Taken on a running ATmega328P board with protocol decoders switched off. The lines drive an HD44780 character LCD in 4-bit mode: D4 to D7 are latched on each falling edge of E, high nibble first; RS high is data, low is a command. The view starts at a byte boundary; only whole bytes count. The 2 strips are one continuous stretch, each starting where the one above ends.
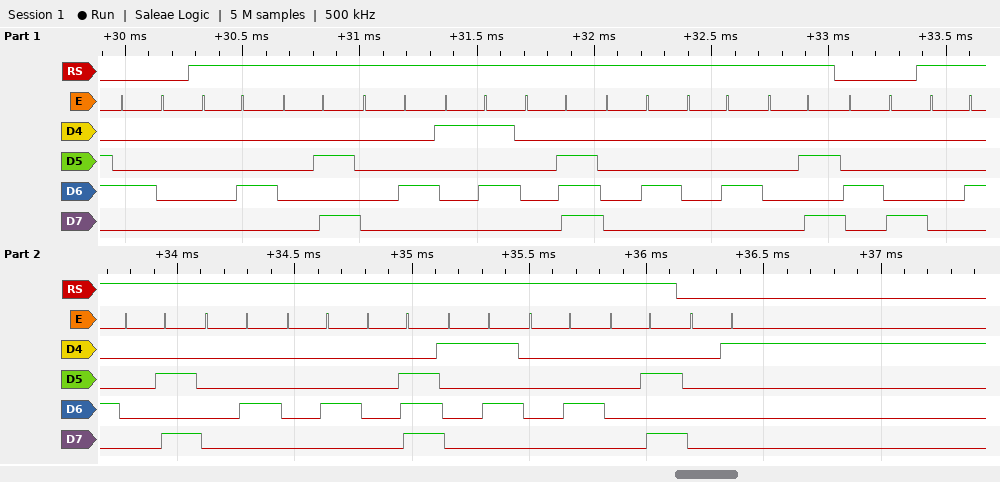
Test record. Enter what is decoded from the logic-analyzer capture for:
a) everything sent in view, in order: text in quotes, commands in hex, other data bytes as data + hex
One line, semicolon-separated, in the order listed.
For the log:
0x40 data 04 0A 04 15 0E 04 04 0A 0x48 data 04 0A 04 04 0E 15 04 0A 0x01
